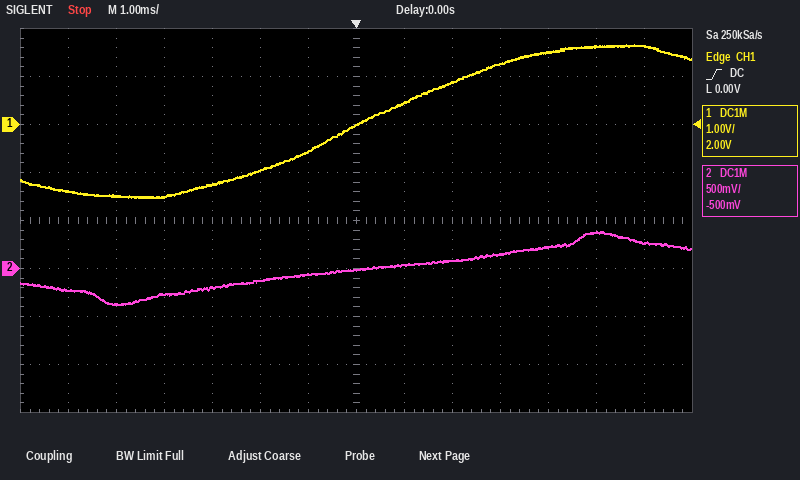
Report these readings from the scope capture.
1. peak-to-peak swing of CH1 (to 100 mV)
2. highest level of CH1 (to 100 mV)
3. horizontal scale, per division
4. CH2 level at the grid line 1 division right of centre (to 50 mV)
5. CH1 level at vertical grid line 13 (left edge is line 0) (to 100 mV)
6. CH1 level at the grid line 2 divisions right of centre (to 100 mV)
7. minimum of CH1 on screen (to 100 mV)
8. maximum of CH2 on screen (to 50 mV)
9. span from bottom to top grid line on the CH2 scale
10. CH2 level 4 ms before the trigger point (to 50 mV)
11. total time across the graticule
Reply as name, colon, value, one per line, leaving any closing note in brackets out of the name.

peak-to-peak swing of CH1: 3.2 V
highest level of CH1: 1.7 V
horizontal scale, per division: 1 ms
CH2 level at the grid line 1 division right of centre: 50 mV
CH1 level at vertical grid line 13 (left edge is line 0): 1.6 V
CH1 level at the grid line 2 divisions right of centre: 900 mV
minimum of CH1 on screen: -1.5 V
maximum of CH2 on screen: 400 mV
span from bottom to top grid line on the CH2 scale: 4 V
CH2 level 4 ms before the trigger point: -250 mV
total time across the graticule: 14 ms
